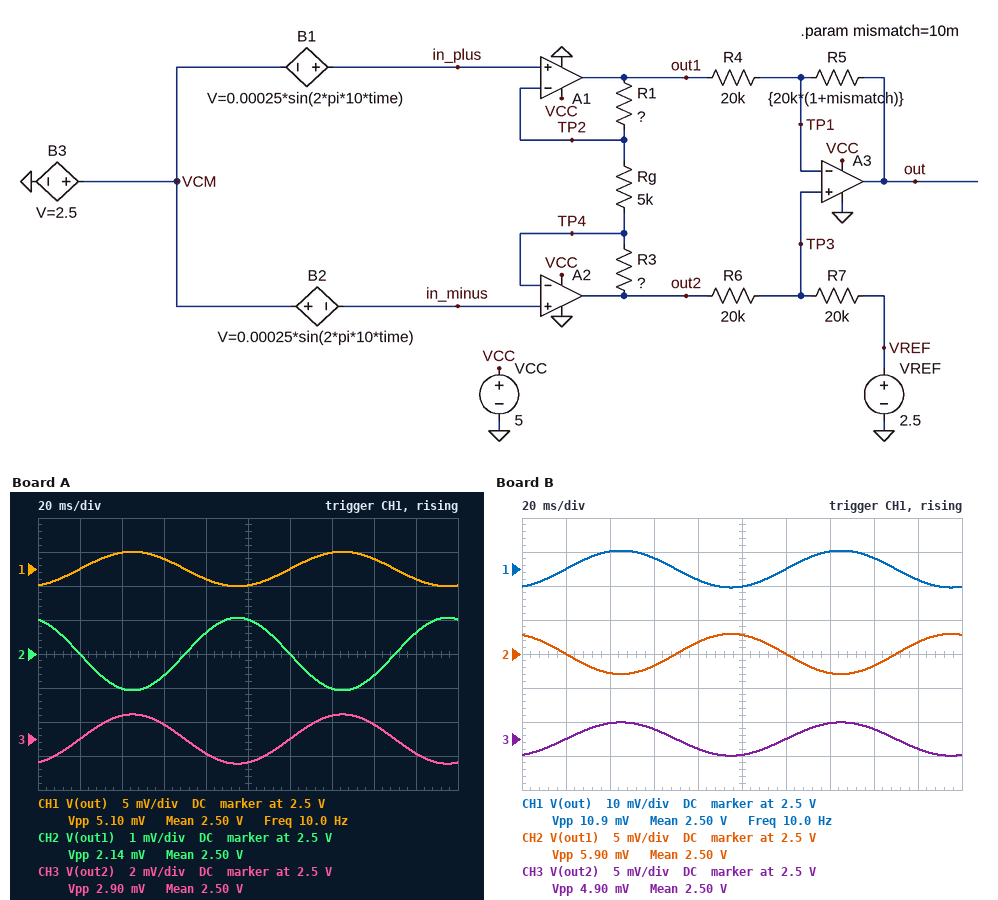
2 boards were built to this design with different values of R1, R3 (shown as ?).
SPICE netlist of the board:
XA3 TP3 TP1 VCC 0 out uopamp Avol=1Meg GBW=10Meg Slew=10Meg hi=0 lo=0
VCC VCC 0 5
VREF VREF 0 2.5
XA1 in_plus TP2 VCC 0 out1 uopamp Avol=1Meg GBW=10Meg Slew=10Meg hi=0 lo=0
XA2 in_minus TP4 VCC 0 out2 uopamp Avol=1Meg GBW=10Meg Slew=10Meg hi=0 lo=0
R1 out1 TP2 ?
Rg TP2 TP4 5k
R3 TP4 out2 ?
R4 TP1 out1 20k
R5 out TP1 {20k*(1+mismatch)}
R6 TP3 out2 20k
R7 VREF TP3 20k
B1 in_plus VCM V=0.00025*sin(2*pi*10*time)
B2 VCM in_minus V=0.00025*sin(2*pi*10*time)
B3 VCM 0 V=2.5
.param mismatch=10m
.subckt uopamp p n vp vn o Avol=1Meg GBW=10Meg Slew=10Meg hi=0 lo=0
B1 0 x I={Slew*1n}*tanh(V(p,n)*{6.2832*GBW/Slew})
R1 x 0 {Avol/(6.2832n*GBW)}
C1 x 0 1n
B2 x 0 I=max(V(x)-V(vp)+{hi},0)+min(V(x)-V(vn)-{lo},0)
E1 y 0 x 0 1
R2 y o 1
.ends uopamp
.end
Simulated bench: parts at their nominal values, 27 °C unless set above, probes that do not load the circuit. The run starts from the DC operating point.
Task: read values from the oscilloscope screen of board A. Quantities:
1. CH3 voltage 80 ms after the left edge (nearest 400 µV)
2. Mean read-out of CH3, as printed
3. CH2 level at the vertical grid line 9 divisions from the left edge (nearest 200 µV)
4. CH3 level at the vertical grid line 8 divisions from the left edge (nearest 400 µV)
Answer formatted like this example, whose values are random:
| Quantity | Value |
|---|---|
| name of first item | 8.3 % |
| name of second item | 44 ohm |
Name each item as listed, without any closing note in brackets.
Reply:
| Quantity | Value |
|---|---|
| CH3 voltage 80 ms after the left edge | 2.4992 V |
| Mean read-out of CH3, as printed | 2.50 V |
| CH2 level at the vertical grid line 9 divisions from the left edge | 2.5006 V |
| CH3 level at the vertical grid line 8 divisions from the left edge | 2.5008 V |
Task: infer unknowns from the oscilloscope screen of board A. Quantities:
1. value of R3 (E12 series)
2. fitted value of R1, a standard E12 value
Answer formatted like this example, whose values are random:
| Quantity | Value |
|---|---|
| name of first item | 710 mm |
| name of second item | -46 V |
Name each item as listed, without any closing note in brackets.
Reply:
| Quantity | Value |
|---|---|
| value of R3 | 12 kΩ |
| fitted value of R1, a standard E12 value | 8.2 kΩ |
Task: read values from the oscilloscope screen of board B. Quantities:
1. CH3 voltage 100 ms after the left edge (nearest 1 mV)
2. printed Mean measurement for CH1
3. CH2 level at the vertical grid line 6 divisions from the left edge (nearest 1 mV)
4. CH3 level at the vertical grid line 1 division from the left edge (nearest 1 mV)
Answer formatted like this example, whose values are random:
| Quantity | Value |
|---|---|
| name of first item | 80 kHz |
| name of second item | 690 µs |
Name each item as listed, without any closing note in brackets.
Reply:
| Quantity | Value |
|---|---|
| CH3 voltage 100 ms after the left edge | 2.498 V |
| printed Mean measurement for CH1 | 2.50 V |
| CH2 level at the vertical grid line 6 divisions from the left edge | 2.500 V |
| CH3 level at the vertical grid line 1 division from the left edge | 2.500 V |
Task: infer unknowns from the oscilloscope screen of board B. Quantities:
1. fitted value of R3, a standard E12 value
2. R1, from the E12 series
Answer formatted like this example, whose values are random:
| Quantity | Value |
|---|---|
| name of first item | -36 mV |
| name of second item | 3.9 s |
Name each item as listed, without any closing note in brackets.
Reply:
| Quantity | Value |
|---|---|
| fitted value of R3, a standard E12 value | 22 kΩ |
| R1, from the E12 series | 27 kΩ |
